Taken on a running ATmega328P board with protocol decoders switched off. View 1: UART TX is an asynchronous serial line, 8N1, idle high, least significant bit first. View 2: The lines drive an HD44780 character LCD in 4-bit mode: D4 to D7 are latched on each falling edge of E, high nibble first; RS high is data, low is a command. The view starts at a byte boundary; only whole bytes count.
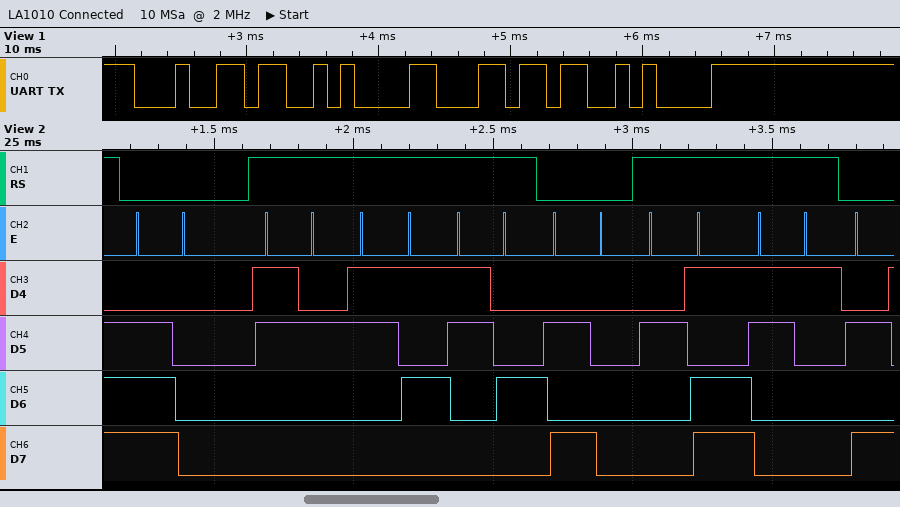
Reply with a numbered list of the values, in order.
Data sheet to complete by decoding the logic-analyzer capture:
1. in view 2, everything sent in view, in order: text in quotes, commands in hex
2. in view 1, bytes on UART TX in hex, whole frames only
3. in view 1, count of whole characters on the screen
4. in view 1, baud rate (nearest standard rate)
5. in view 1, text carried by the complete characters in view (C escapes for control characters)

1. 0xE0 "254" 0xA0 "-1"
2. 64 0A 6C 0A
3. 4
4. 9600 baud
5. "d\nl\n"
